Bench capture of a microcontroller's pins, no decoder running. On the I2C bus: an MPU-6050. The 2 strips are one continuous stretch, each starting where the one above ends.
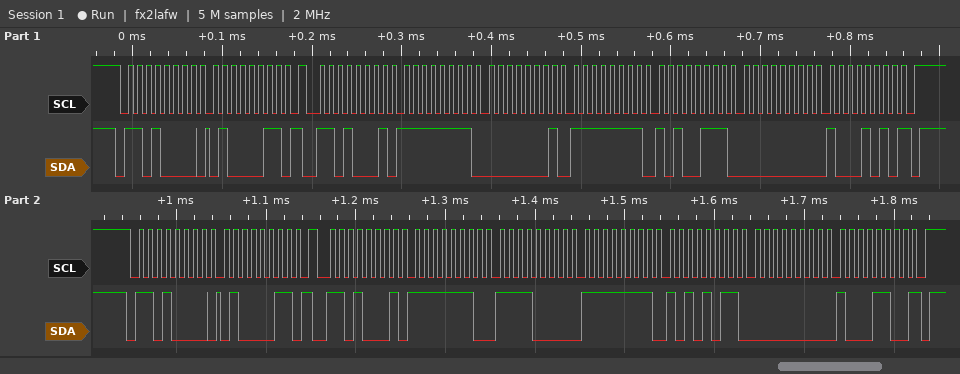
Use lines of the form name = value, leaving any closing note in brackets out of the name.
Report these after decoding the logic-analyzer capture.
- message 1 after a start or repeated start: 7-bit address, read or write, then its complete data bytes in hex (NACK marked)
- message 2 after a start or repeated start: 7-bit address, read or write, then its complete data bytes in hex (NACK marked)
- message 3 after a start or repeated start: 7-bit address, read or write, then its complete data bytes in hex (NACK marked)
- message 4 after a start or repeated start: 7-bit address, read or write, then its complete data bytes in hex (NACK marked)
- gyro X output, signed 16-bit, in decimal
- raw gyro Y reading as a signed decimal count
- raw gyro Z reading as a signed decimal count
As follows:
message 1 after a start or repeated start: 7-bit address, read or write, then its complete data bytes in hex = 0x68 write: 43
message 2 after a start or repeated start: 7-bit address, read or write, then its complete data bytes in hex = 0x68 read: FF 01 FF A7 00 8A NACK
message 3 after a start or repeated start: 7-bit address, read or write, then its complete data bytes in hex = 0x68 write: 43
message 4 after a start or repeated start: 7-bit address, read or write, then its complete data bytes in hex = 0x68 read: FE F0 FF AB 00 8C NACK
gyro X output, signed 16-bit, in decimal = -255
raw gyro Y reading as a signed decimal count = -89
raw gyro Z reading as a signed decimal count = 138
